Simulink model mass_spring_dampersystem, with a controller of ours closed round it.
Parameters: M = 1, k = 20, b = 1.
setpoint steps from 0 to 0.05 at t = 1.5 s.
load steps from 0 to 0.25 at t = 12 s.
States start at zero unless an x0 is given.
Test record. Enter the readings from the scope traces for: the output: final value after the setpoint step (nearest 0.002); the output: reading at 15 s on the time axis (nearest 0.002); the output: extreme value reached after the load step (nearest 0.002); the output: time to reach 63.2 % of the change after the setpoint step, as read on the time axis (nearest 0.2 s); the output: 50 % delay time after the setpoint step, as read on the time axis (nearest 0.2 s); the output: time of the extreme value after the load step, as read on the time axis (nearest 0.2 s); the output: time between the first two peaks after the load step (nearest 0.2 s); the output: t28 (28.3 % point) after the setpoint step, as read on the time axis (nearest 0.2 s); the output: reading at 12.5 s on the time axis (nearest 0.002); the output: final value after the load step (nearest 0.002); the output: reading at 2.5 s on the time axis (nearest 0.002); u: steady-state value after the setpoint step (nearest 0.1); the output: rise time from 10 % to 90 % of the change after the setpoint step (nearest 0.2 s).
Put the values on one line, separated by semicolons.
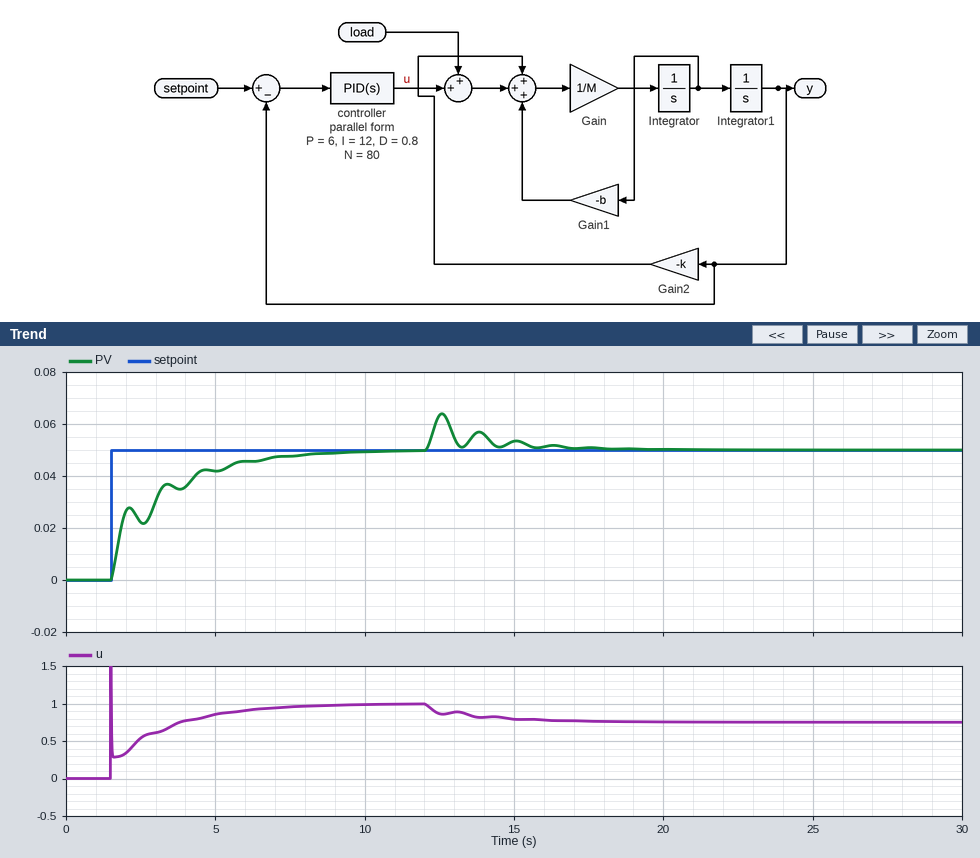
0.050; 0.054; 0.064; 3.0 s; 2.0 s; 12.6 s; 1.2 s; 1.8 s; 0.064; 0.050; 0.022; 1.0; 4.0 s
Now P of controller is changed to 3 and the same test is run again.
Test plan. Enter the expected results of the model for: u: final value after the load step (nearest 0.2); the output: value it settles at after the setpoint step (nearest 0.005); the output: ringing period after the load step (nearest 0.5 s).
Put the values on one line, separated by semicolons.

0.8; 0.050; 1.5 s
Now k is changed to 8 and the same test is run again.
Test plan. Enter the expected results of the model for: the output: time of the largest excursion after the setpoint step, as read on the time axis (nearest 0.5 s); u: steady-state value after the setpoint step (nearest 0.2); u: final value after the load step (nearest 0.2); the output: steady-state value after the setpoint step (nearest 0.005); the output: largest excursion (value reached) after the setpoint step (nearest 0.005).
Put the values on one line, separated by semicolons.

4.0 s; 0.4; 0.2; 0.050; 0.055
